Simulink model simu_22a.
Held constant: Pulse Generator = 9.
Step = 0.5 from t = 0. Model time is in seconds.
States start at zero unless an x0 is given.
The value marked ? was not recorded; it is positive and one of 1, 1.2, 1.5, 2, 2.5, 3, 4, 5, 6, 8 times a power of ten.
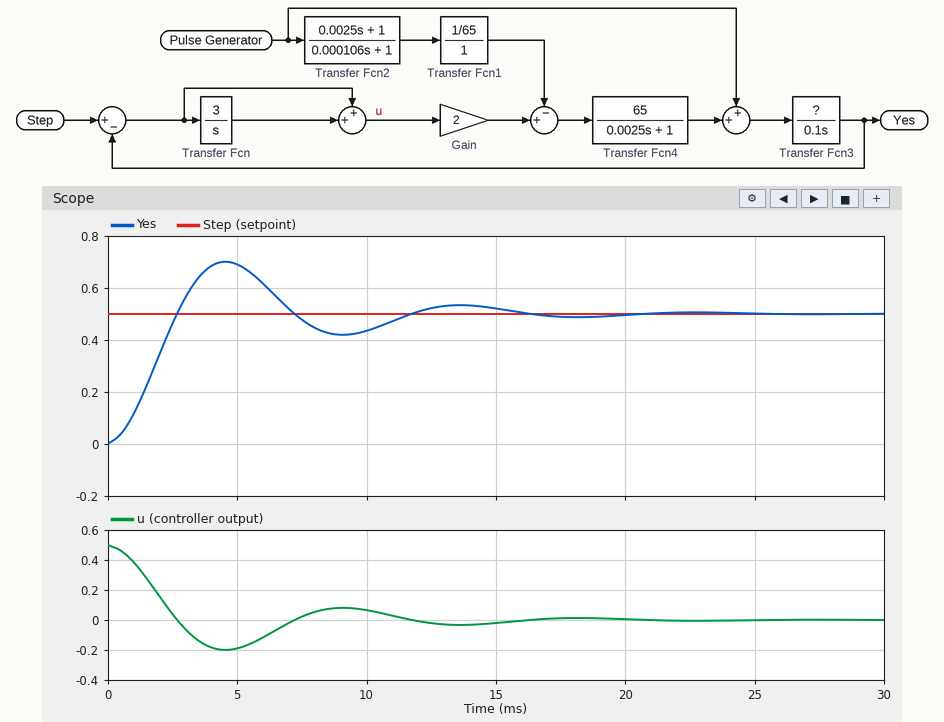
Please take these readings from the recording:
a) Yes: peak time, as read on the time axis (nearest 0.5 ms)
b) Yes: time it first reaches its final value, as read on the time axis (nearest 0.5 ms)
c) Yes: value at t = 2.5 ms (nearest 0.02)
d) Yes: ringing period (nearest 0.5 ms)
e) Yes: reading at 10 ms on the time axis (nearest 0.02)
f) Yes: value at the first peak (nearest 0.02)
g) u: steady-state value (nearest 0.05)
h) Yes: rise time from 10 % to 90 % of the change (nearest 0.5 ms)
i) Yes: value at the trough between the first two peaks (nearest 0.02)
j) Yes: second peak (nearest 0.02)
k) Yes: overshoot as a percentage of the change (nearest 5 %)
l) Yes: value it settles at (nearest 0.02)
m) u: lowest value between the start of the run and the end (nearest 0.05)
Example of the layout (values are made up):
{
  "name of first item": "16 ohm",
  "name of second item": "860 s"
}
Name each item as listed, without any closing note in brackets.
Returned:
{
  "Yes: peak time, as read on the time axis": "4.5 ms",
  "Yes: time it first reaches its final value, as read on the time axis": "2.5 ms",
  "Yes: value at t = 2.5 ms": "0.46",
  "Yes: ringing period": "9.0 ms",
  "Yes: reading at 10 ms on the time axis": "0.44",
  "Yes: value at the first peak": "0.70",
  "u: steady-state value": "0.00",
  "Yes: rise time from 10 % to 90 % of the change": "2.0 ms",
  "Yes: value at the trough between the first two peaks": "0.42",
  "Yes: second peak": "0.54",
  "Yes: overshoot as a percentage of the change": "40 %",
  "Yes: value it settles at": "0.50",
  "u: lowest value between the start of the run and the end": "-0.20"
}
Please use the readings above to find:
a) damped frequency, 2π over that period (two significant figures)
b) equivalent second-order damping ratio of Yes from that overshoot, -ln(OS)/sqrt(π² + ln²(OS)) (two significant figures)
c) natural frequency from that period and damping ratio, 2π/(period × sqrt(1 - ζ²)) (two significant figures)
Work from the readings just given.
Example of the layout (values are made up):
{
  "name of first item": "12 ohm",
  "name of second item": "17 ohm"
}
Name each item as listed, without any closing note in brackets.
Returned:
{
  "damped frequency, 2π over that period": "0.70 rad/ms",
  "equivalent second-order damping ratio of Yes from that overshoot, -ln(OS)/sqrt(π² + ln²(OS))": "0.28",
  "natural frequency from that period and damping ratio, 2π/(period × sqrt(1 - ζ²))": "0.73 rad/ms"
}
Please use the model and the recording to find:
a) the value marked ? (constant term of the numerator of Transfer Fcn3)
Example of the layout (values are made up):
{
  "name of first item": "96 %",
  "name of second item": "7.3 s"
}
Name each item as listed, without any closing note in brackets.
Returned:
{
  "the value marked ?": "1"
}
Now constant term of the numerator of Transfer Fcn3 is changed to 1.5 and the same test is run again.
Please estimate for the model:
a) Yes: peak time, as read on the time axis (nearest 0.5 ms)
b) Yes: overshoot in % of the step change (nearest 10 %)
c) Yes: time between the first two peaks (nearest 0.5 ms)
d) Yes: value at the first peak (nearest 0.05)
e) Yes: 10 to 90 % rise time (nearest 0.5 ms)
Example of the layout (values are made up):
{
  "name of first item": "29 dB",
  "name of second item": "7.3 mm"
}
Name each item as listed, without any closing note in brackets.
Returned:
{
  "Yes: peak time, as read on the time axis": "3.5 ms",
  "Yes: overshoot in % of the step change": "50 %",
  "Yes: time between the first two peaks": "7.5 ms",
  "Yes: value at the first peak": "0.75",
  "Yes: 10 to 90 % rise time": "1.5 ms"
}
